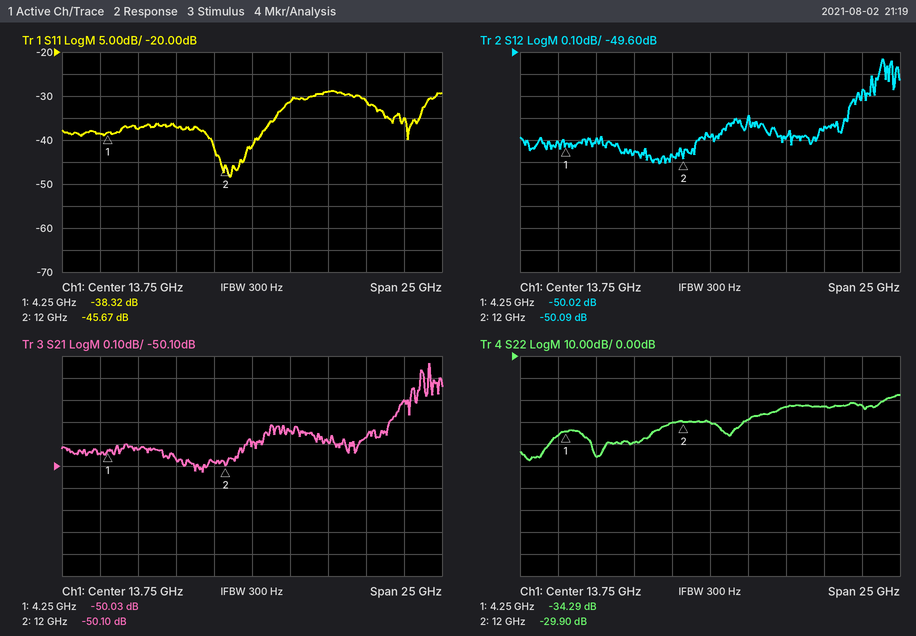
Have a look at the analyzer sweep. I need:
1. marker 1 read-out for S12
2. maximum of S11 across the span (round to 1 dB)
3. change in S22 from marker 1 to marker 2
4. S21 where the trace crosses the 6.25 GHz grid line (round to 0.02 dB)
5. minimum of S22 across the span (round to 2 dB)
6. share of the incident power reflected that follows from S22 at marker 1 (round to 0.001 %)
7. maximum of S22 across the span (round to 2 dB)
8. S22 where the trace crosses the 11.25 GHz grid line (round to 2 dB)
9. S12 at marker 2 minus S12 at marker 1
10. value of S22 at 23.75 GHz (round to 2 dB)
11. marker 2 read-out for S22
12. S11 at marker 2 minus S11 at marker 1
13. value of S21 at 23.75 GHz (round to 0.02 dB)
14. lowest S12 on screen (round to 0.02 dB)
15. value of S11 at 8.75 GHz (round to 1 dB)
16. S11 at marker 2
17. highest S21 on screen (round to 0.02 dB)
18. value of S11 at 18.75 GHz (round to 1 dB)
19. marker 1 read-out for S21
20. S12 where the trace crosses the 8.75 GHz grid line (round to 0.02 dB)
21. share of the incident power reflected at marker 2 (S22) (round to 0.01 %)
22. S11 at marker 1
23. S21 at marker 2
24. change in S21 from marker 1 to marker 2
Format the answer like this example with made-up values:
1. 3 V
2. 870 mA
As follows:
1. -50.02 dB
2. -29 dB
3. 4.39 dB
4. -50.02 dB
5. -48 dB
6. 0.037 %
7. -18 dB
8. -30 dB
9. -0.07 dB
10. -22 dB
11. -29.90 dB
12. -7.35 dB
13. -49.80 dB
14. -50.10 dB
15. -37 dB
16. -45.67 dB
17. -49.64 dB
18. -29 dB
19. -50.03 dB
20. -50.06 dB
21. 0.10 %
22. -38.32 dB
23. -50.10 dB
24. -0.07 dB
